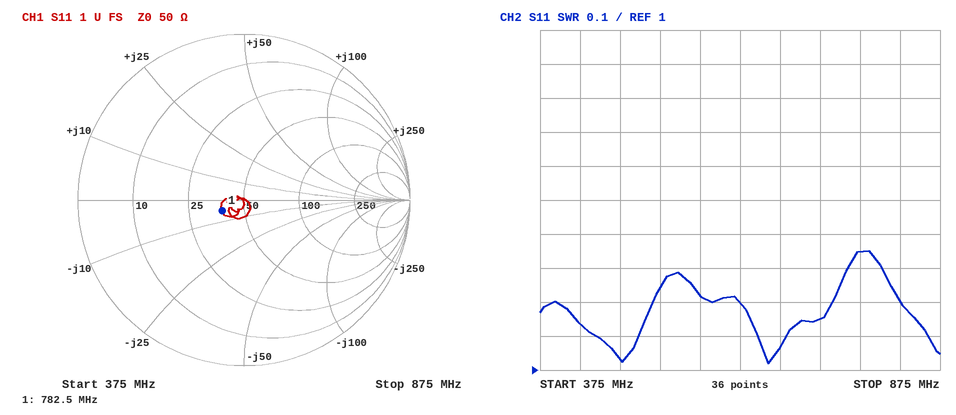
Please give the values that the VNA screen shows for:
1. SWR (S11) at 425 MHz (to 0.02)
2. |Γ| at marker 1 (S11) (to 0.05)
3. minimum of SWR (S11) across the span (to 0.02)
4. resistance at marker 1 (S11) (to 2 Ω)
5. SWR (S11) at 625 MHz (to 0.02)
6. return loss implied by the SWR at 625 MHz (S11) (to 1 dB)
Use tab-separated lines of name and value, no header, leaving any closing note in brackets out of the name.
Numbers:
SWR (S11) at 425 MHz	1.14
|Γ| at marker 1 (S11)	0.15
minimum of SWR (S11) across the span	1.02
resistance at marker 1 (S11)	38 Ω
SWR (S11) at 625 MHz	1.20
return loss implied by the SWR at 625 MHz (S11)	21 dB
